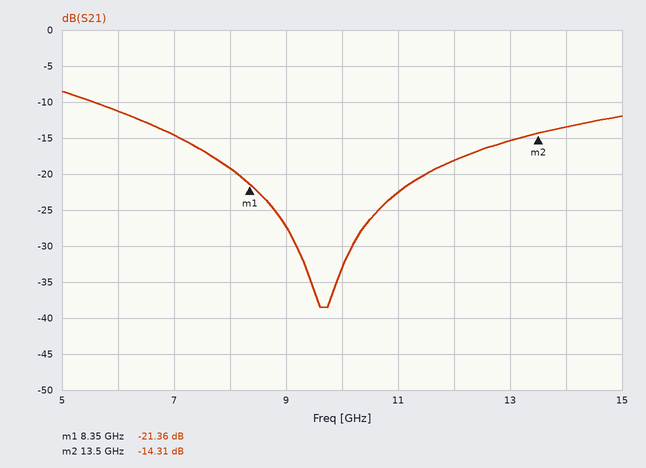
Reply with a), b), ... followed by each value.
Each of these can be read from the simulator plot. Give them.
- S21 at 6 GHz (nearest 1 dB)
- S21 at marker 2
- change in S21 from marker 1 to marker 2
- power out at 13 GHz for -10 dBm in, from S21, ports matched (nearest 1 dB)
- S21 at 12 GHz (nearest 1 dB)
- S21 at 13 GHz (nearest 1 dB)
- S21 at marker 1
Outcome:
a) -11 dB
b) -14.31 dB
c) 7.05 dB
d) -25 dBm
e) -18 dB
f) -15 dB
g) -21.36 dB
